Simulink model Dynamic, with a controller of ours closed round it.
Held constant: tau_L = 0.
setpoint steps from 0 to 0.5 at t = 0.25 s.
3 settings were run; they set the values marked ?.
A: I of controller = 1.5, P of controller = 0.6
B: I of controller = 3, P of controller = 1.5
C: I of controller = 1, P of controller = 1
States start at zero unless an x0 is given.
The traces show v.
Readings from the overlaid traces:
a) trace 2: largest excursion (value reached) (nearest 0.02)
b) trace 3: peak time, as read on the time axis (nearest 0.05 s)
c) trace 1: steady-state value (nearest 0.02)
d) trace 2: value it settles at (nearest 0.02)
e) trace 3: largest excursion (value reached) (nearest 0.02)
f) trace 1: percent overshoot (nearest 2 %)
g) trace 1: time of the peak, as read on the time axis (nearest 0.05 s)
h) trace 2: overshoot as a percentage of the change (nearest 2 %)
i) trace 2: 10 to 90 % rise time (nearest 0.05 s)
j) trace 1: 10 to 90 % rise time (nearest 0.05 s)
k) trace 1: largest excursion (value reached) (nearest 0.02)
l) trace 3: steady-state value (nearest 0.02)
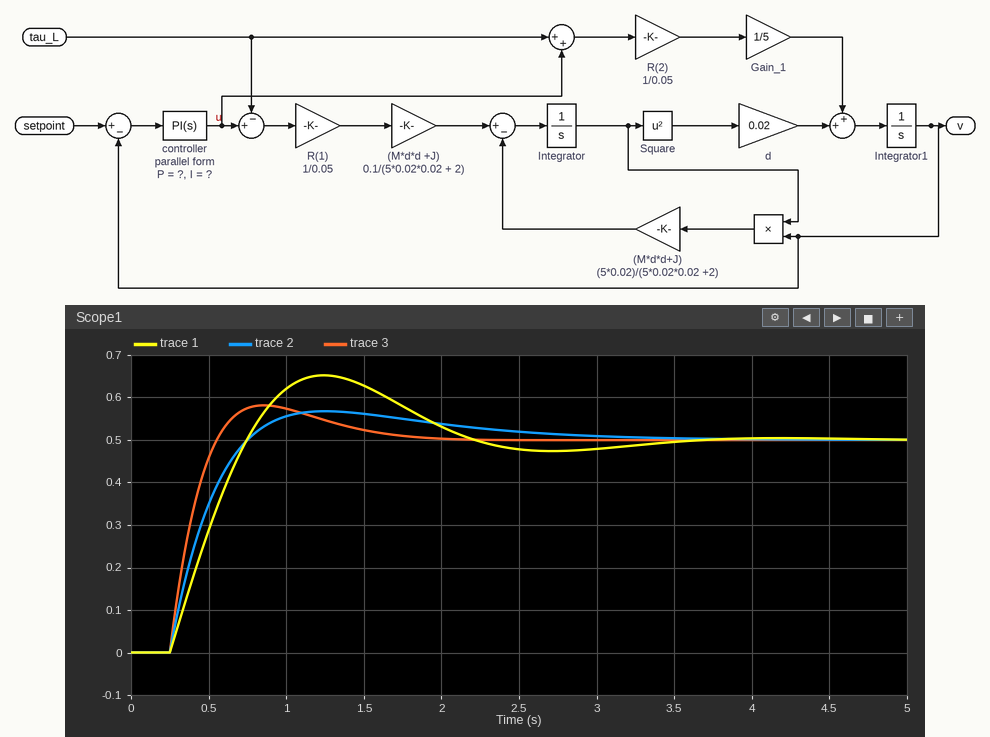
0.56
0.85 s
0.50
0.50
0.58
30 %
1.25 s
14 %
0.35 s
0.40 s
0.66
0.50
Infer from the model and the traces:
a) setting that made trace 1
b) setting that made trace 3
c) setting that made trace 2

A
B
C
